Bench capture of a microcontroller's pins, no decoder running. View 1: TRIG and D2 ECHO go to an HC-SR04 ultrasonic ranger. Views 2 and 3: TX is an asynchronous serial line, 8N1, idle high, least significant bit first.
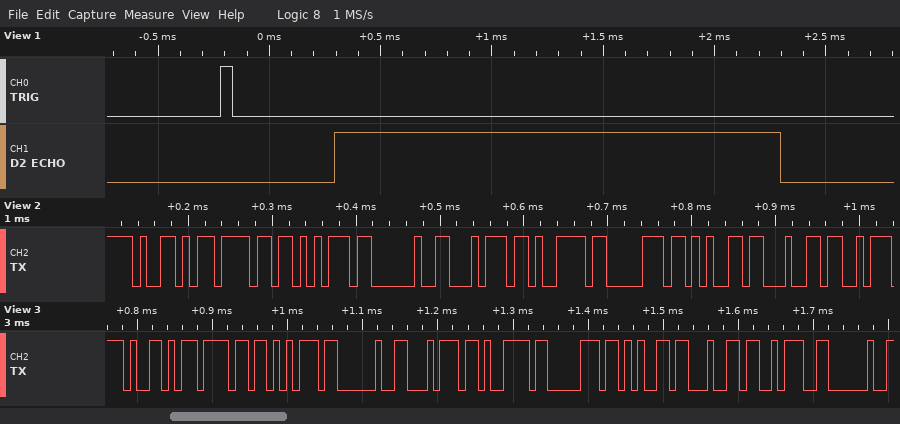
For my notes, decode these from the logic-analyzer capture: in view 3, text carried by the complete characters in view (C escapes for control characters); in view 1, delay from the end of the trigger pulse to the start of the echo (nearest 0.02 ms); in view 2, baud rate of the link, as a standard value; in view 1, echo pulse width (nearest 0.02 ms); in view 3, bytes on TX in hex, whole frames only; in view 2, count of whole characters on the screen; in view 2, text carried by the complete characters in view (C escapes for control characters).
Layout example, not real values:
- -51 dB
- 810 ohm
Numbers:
- "You typed: "
- 0.46 ms
- 115200 baud
- 2.00 ms
- 0x59 0x6F 0x75 0x20 0x74 0x79 0x70 0x65 0x64 0x3A 0x20
- 9
- "You typed"
